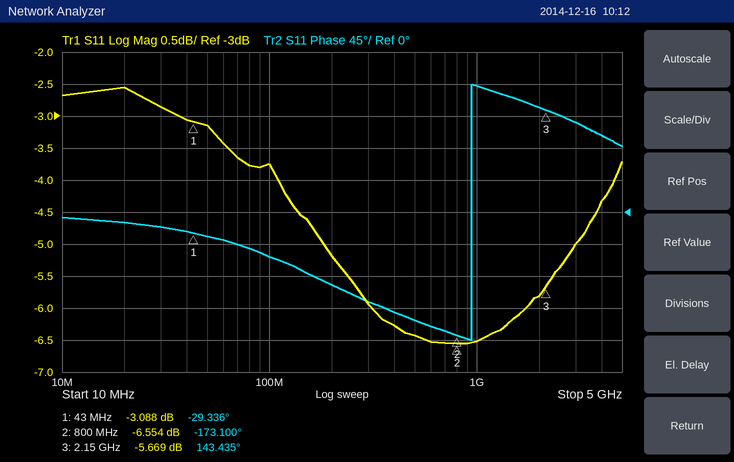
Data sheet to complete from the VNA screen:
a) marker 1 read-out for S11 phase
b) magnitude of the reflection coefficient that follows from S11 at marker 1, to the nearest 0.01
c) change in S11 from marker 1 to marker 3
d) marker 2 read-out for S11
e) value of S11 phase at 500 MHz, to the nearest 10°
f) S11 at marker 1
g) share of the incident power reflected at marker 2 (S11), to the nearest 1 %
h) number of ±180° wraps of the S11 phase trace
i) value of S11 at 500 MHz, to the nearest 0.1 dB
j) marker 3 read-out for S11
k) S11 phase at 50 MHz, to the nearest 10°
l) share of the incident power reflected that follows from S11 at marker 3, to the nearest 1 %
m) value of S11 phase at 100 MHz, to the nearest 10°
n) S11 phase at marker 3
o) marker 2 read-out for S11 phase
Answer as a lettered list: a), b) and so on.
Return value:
a) -29.336°
b) 0.70
c) -2.581 dB
d) -6.554 dB
e) -150°
f) -3.088 dB
g) 22 %
h) 1
i) -6.4 dB
j) -5.669 dB
k) -30°
l) 27 %
m) -60°
n) 143.435°
o) -173.100°
